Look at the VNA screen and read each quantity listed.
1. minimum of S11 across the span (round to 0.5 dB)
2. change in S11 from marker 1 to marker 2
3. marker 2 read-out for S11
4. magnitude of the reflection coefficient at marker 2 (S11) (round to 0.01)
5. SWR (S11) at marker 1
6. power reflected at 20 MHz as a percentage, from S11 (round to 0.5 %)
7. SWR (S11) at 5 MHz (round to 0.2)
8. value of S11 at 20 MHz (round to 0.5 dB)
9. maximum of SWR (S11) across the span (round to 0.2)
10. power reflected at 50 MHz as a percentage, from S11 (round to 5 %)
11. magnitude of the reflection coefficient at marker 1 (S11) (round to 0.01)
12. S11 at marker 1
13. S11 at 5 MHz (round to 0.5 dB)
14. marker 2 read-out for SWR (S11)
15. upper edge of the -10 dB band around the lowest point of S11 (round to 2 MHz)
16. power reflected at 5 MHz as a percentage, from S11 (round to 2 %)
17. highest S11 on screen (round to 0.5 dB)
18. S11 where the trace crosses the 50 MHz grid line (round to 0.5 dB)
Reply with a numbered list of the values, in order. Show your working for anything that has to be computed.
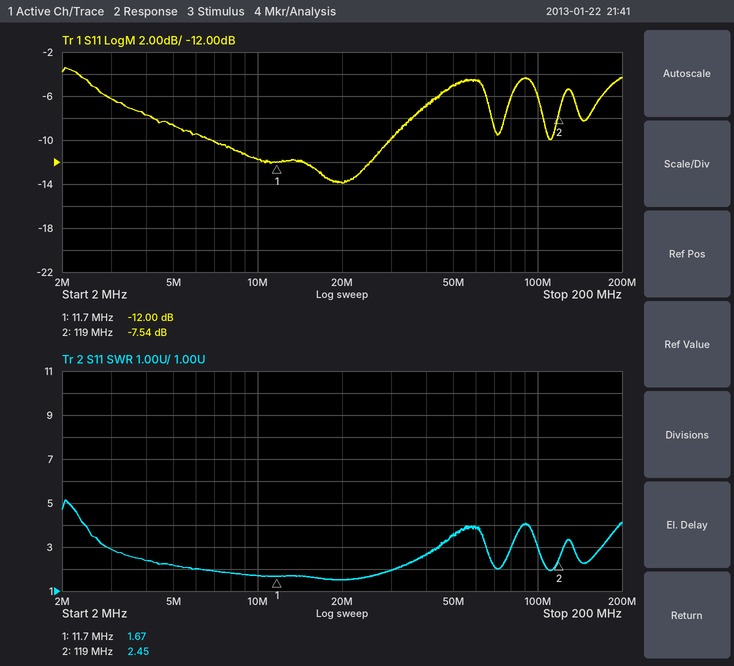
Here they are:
1. -14.0 dB
2. -7.54 − (-12) = 4.46 dB
3. -7.54 dB
4. 10^(-7.54/20) ≈ 0.42
5. 1.67
6. 10^(-14/10) ≈ 4.0 %
7. 2.2
8. -14.0 dB
9. 5.2
10. 10^(-5/10) ≈ 31.6 %, so 30 % to the nearest 5 %
11. 10^(-12/20) ≈ 0.25
12. -12.00 dB
13. -8.5 dB
14. 2.45
15. 30 MHz
16. 10^(-8.5/10) ≈ 14 %
17. -3.5 dB
18. -5.0 dB
